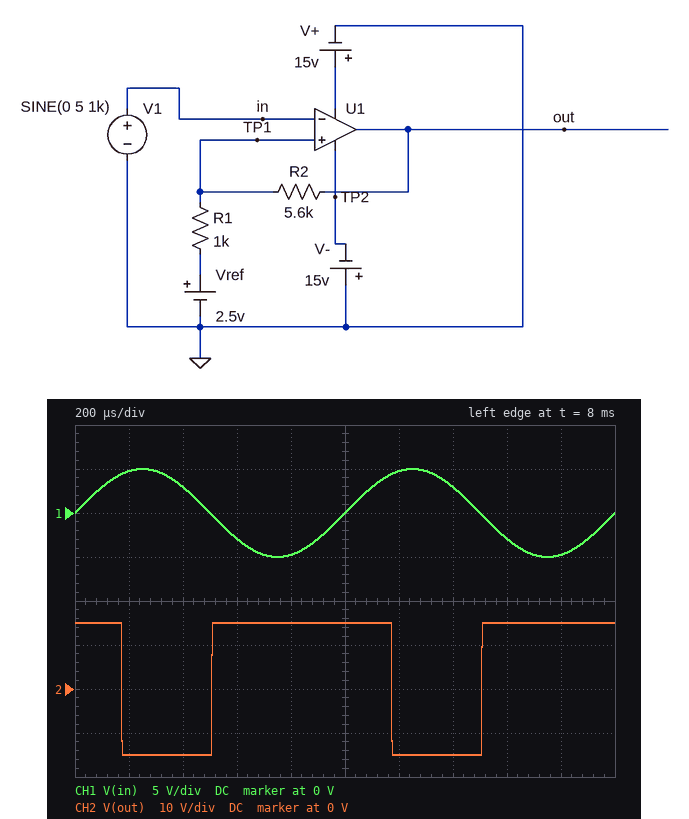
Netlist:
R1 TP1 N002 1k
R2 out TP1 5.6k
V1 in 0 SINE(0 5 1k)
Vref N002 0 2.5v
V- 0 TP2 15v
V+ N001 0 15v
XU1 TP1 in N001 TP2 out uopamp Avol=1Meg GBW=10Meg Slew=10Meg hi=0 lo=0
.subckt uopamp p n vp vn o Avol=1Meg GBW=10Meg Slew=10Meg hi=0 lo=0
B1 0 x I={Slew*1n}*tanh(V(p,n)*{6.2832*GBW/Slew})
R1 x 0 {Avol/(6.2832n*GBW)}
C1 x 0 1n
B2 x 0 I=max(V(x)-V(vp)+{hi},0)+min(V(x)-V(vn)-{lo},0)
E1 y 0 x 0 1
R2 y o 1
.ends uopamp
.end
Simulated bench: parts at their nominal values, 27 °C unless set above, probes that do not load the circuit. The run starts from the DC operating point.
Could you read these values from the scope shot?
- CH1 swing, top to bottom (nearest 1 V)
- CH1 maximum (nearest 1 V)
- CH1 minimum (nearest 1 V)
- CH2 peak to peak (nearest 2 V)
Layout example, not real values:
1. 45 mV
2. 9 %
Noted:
1. 10 V
2. 5 V
3. -5 V
4. 30 V
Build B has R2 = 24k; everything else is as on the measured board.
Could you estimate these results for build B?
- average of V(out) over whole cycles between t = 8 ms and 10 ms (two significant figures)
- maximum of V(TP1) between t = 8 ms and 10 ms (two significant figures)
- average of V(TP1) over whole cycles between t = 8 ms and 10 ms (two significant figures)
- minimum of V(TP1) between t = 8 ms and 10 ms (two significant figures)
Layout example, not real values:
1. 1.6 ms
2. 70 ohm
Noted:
1. 4.8 V
2. 3.0 V
3. 2.6 V
4. 1.8 V
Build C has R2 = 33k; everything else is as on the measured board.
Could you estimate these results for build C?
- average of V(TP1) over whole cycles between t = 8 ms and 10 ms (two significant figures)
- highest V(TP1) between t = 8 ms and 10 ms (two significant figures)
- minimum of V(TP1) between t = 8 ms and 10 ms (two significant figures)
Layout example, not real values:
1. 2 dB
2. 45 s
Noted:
1. 2.6 V
2. 2.9 V
3. 2.0 V
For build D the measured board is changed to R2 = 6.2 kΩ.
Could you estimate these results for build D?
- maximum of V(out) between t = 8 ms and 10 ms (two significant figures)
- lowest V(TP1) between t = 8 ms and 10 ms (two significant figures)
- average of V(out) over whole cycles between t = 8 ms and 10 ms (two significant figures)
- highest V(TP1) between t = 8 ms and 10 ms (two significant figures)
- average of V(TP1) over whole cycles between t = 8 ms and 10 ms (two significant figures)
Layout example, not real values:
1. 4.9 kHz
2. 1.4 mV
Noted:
1. 15 V
2. 68 mV
3. 4.9 V
4. 4.2 V
5. 2.8 V
